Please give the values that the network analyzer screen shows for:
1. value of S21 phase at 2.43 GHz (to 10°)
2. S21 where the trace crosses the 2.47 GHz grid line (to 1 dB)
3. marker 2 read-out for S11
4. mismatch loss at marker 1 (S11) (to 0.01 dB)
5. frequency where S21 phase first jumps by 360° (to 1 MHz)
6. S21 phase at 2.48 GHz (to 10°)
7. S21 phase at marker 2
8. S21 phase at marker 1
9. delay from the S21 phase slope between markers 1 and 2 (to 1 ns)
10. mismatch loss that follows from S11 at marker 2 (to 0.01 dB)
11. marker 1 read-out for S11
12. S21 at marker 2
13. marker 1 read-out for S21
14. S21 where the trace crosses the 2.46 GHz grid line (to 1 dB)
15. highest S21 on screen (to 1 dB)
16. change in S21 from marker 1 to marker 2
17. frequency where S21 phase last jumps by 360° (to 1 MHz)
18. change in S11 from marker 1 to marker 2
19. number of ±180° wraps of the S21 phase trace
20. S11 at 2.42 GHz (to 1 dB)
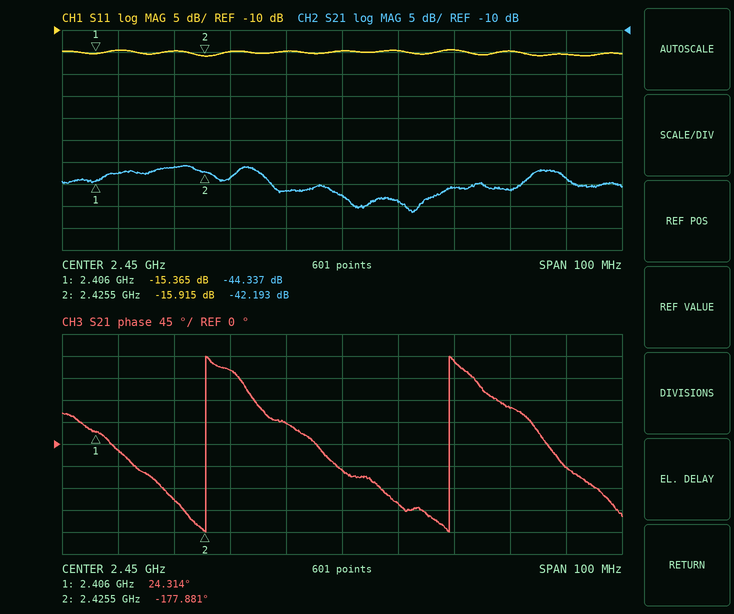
150°
-46 dB
-15.915 dB
0.13 dB
2.426 GHz
70°
-177.881°
24.314°
29 ns
0.11 dB
-15.365 dB
-42.193 dB
-44.337 dB
-49 dB
-41 dB
2.144 dB
2.469 GHz
-0.550 dB
2
-15 dB
